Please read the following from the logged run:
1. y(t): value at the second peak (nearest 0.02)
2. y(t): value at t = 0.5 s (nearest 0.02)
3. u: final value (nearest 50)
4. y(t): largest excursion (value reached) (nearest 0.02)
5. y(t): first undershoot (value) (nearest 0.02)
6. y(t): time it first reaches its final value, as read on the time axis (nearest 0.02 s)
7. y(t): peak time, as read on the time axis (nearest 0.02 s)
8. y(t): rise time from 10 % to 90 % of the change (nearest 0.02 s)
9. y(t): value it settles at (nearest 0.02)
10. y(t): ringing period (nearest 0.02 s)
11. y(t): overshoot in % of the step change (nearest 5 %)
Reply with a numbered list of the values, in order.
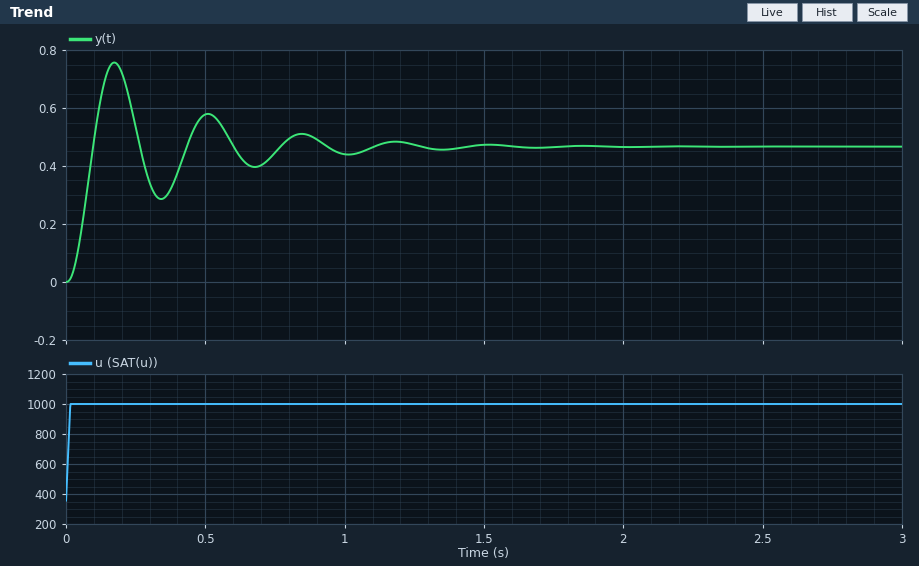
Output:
1. 0.58
2. 0.58
3. 1000
4. 0.76
5. 0.28
6. 0.10 s
7. 0.18 s
8. 0.06 s
9. 0.46
10. 0.34 s
11. 60 %
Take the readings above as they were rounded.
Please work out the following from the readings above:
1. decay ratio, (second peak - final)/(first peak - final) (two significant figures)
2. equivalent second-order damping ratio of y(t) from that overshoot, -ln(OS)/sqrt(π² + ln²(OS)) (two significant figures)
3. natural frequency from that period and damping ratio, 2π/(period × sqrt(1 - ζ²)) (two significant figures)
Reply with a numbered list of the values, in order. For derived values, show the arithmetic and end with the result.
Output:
1. (0.58 - 0.46) / (0.76 - 0.46) = 0.40
2. ln(0.6) = -0.511; 0.511 / sqrt(9.870 + 0.261) = 0.16
3. 2π / (0.34 × sqrt(1 - 0.16²)) = 19 rad/s
